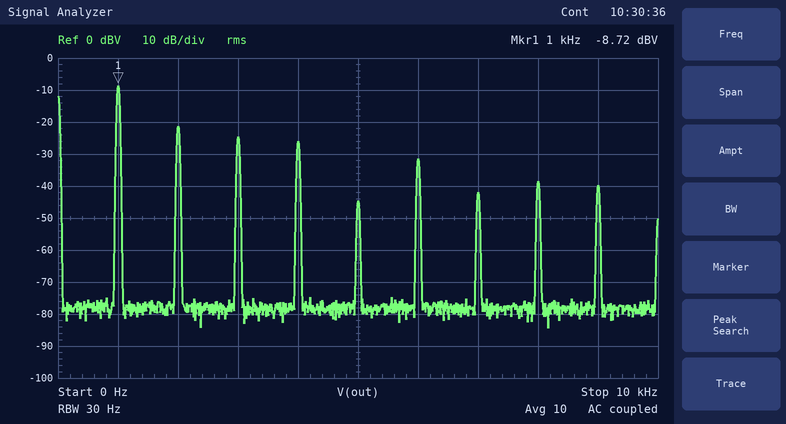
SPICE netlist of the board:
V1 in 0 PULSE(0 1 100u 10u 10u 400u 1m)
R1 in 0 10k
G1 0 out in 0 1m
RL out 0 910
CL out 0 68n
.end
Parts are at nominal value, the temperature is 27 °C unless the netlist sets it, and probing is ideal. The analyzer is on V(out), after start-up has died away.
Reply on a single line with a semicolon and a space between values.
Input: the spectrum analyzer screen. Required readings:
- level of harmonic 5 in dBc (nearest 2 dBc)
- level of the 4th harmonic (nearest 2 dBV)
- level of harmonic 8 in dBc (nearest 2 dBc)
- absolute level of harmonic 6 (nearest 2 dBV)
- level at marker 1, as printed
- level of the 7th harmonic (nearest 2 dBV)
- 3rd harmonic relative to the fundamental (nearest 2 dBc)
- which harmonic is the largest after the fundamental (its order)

-36 dBc; -26 dBV; -30 dBc; -32 dBV; -8.72 dBV; -42 dBV; -16 dBc; 2
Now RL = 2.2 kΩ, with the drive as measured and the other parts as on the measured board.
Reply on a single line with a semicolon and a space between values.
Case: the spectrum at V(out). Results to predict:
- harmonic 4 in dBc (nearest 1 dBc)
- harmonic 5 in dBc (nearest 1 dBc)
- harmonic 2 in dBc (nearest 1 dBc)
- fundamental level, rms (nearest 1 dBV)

-22 dBc; -41 dBc; -15 dBc; -3 dBV
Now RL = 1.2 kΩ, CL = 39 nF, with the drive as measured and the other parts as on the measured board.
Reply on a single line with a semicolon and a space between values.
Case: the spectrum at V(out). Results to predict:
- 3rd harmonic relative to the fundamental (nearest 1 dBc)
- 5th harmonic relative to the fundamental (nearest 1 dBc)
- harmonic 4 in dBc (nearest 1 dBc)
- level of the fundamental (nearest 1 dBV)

-15 dBc; -34 dBc; -16 dBc; -6 dBV
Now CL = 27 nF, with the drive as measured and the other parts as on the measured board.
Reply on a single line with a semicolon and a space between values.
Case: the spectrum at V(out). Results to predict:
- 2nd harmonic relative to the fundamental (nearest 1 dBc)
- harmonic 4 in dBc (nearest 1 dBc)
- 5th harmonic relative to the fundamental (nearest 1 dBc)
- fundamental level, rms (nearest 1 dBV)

-11 dBc; -14 dBc; -32 dBc; -8 dBV
